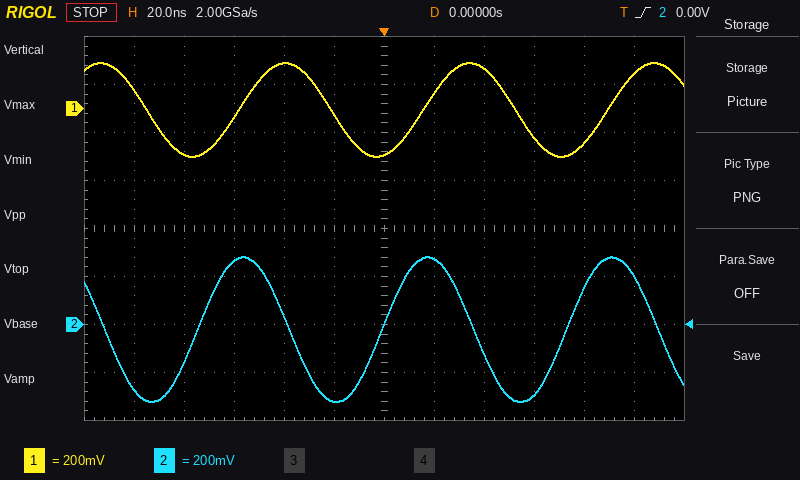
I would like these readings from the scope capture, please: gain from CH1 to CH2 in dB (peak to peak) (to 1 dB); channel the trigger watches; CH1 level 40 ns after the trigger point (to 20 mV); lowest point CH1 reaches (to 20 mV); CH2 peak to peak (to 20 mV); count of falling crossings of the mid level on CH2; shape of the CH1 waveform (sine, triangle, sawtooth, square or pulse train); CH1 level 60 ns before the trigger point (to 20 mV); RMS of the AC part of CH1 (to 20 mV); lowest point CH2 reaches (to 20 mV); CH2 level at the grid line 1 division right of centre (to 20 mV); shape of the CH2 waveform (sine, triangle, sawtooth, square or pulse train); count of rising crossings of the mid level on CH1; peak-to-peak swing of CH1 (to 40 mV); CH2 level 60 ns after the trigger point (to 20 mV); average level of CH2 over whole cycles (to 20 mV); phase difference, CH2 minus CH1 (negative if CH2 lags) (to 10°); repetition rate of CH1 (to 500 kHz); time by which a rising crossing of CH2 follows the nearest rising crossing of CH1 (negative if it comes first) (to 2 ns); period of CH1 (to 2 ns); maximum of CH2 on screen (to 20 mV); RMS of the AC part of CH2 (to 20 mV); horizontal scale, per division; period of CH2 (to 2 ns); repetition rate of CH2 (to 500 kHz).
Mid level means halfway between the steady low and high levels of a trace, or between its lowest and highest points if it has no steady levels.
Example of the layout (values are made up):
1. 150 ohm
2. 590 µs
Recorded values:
1. 4 dB
2. CH2
3. 160 mV
4. -200 mV
5. 600 mV
6. 4
7. sine
8. -40 mV
9. 140 mV
10. -320 mV
11. 280 mV
12. sine
13. 3
14. 400 mV
15. -300 mV
16. -20 mV
17. +80°
18. 13.5 MHz
19. -16 ns
20. 74 ns
21. 280 mV
22. 220 mV
23. 20 ns
24. 74 ns
25. 13.5 MHz
